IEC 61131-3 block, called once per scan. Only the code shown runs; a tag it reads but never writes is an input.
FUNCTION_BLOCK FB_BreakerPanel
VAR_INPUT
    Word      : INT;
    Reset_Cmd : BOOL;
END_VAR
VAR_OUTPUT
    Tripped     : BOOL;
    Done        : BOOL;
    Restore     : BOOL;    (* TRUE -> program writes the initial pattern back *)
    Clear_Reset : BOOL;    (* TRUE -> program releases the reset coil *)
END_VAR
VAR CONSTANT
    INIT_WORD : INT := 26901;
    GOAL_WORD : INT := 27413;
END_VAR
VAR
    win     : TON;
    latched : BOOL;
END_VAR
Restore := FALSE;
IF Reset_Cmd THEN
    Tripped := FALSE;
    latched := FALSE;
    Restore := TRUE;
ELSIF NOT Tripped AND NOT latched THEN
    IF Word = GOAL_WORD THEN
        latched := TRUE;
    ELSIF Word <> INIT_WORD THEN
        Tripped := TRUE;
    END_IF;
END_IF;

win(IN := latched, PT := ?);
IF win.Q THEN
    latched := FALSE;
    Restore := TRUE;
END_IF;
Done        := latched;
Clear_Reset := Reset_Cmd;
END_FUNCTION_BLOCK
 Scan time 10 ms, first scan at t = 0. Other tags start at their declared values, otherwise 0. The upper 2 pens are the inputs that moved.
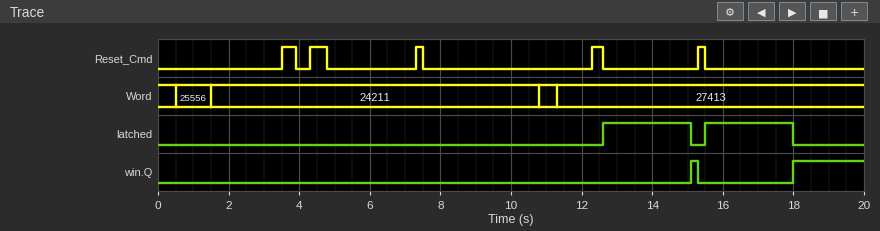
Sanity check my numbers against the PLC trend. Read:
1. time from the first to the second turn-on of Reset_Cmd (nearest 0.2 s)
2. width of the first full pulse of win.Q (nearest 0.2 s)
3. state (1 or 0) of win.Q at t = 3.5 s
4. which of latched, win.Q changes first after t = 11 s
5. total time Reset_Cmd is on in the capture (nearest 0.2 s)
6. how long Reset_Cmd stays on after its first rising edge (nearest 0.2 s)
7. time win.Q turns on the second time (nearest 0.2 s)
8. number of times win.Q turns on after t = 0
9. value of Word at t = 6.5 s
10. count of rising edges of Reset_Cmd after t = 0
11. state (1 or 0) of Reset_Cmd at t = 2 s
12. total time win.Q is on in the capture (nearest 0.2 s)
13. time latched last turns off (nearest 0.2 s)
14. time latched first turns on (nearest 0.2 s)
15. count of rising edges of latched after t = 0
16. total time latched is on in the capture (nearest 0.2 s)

0.8 s
0.2 s
0
latched
1.6 s
0.4 s
18.0 s
2
24211
5
0
2.2 s
18.0 s
12.6 s
2
5.0 s
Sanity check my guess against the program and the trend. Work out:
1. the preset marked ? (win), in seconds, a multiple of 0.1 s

2.5 s
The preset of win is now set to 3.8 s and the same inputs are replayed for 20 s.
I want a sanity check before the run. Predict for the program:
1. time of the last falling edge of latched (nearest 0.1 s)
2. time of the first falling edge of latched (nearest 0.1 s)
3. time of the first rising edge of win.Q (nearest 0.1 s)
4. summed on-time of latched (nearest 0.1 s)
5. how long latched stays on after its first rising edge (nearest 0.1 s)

19.3 s
15.3 s
19.3 s
6.5 s
2.7 s
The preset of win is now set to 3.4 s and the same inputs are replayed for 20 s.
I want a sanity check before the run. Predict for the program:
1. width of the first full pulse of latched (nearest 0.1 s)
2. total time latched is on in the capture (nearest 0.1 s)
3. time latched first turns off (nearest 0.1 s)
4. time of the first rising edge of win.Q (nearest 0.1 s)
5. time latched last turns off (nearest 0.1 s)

2.7 s
6.1 s
15.3 s
18.9 s
18.9 s
